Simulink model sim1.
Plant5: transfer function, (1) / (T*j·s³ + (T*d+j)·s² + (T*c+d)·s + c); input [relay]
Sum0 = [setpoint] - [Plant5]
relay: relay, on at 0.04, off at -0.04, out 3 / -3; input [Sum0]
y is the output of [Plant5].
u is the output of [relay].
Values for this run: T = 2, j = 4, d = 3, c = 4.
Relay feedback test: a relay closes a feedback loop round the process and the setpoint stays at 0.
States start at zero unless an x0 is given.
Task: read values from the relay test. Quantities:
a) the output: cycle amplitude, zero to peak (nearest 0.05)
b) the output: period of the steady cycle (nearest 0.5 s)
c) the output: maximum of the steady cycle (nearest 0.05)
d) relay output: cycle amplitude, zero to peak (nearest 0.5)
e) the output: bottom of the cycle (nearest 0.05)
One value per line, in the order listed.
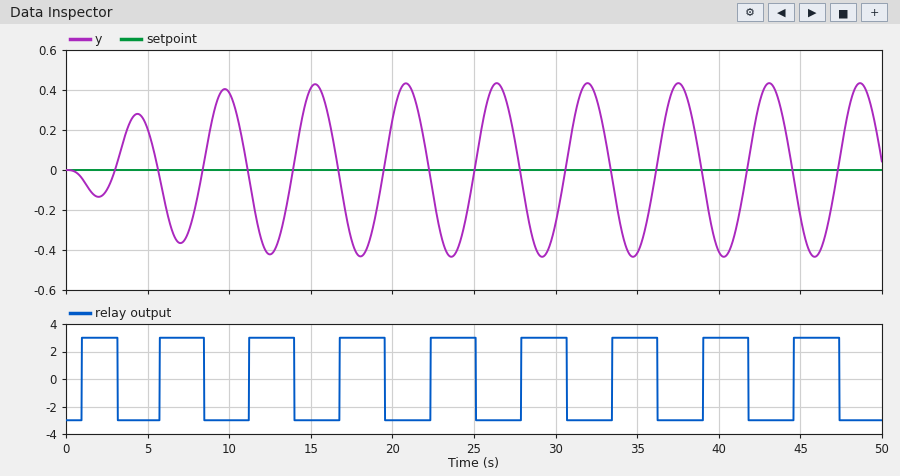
0.45
5.5 s
0.45
3.0
-0.45
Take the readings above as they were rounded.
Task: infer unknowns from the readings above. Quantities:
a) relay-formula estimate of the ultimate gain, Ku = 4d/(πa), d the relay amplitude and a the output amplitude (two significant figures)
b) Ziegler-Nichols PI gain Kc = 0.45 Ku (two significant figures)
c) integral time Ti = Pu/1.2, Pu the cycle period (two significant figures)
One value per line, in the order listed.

8.5
3.8
4.6 s
